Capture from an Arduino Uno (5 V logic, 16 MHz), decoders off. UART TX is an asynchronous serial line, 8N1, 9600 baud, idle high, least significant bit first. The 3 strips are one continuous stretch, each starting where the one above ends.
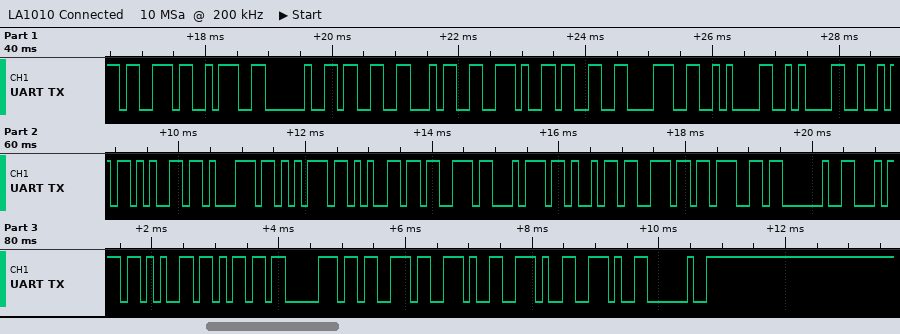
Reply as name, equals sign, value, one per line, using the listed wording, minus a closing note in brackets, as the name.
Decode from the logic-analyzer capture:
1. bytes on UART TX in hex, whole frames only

bytes on UART TX in hex, whole frames only = 0x73 0x3A 0x20 0x33 0x34 0x2E 0x33 0x38 0x0A 0x0A 0x52 0x65 0x71 0x75 0x65 0x73 0x74 0x69 0x6E 0x67 0x20 0x74 0x65 0x6D 0x70 0x73 0x2E 0x2E 0x2E 0x20
